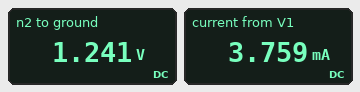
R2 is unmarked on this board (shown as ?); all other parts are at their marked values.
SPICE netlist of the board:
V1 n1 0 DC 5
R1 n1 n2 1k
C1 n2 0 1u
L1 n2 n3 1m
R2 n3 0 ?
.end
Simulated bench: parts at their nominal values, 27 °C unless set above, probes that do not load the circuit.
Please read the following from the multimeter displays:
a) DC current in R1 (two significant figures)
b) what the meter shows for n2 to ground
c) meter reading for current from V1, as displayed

3.8 mA
1.241 V
3.759 mA
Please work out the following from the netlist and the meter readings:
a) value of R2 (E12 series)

330 Ω
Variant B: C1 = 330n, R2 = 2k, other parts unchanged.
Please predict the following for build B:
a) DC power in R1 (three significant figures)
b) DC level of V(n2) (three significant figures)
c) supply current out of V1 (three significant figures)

2.78 mW
3.33 V
1.67 mA
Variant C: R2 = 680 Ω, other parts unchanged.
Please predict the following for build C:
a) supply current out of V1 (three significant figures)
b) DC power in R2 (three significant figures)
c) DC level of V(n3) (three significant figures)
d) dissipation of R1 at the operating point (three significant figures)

2.98 mA
6.02 mW
2.02 V
8.86 mW
